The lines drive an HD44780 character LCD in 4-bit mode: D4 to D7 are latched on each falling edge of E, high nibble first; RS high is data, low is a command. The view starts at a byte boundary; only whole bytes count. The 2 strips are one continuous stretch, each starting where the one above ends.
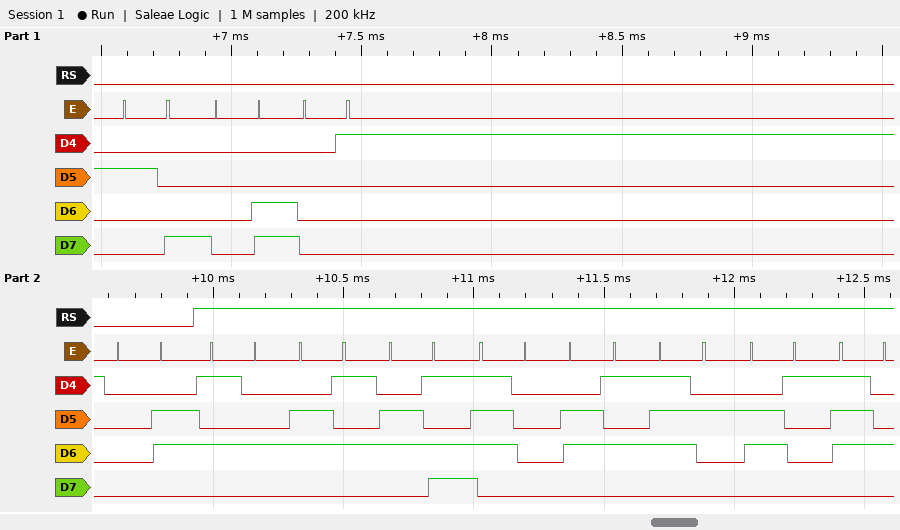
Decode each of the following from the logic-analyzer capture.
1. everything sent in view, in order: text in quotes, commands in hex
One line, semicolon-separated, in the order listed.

0x28 0x0C 0x01 0x06 "Temperat"
